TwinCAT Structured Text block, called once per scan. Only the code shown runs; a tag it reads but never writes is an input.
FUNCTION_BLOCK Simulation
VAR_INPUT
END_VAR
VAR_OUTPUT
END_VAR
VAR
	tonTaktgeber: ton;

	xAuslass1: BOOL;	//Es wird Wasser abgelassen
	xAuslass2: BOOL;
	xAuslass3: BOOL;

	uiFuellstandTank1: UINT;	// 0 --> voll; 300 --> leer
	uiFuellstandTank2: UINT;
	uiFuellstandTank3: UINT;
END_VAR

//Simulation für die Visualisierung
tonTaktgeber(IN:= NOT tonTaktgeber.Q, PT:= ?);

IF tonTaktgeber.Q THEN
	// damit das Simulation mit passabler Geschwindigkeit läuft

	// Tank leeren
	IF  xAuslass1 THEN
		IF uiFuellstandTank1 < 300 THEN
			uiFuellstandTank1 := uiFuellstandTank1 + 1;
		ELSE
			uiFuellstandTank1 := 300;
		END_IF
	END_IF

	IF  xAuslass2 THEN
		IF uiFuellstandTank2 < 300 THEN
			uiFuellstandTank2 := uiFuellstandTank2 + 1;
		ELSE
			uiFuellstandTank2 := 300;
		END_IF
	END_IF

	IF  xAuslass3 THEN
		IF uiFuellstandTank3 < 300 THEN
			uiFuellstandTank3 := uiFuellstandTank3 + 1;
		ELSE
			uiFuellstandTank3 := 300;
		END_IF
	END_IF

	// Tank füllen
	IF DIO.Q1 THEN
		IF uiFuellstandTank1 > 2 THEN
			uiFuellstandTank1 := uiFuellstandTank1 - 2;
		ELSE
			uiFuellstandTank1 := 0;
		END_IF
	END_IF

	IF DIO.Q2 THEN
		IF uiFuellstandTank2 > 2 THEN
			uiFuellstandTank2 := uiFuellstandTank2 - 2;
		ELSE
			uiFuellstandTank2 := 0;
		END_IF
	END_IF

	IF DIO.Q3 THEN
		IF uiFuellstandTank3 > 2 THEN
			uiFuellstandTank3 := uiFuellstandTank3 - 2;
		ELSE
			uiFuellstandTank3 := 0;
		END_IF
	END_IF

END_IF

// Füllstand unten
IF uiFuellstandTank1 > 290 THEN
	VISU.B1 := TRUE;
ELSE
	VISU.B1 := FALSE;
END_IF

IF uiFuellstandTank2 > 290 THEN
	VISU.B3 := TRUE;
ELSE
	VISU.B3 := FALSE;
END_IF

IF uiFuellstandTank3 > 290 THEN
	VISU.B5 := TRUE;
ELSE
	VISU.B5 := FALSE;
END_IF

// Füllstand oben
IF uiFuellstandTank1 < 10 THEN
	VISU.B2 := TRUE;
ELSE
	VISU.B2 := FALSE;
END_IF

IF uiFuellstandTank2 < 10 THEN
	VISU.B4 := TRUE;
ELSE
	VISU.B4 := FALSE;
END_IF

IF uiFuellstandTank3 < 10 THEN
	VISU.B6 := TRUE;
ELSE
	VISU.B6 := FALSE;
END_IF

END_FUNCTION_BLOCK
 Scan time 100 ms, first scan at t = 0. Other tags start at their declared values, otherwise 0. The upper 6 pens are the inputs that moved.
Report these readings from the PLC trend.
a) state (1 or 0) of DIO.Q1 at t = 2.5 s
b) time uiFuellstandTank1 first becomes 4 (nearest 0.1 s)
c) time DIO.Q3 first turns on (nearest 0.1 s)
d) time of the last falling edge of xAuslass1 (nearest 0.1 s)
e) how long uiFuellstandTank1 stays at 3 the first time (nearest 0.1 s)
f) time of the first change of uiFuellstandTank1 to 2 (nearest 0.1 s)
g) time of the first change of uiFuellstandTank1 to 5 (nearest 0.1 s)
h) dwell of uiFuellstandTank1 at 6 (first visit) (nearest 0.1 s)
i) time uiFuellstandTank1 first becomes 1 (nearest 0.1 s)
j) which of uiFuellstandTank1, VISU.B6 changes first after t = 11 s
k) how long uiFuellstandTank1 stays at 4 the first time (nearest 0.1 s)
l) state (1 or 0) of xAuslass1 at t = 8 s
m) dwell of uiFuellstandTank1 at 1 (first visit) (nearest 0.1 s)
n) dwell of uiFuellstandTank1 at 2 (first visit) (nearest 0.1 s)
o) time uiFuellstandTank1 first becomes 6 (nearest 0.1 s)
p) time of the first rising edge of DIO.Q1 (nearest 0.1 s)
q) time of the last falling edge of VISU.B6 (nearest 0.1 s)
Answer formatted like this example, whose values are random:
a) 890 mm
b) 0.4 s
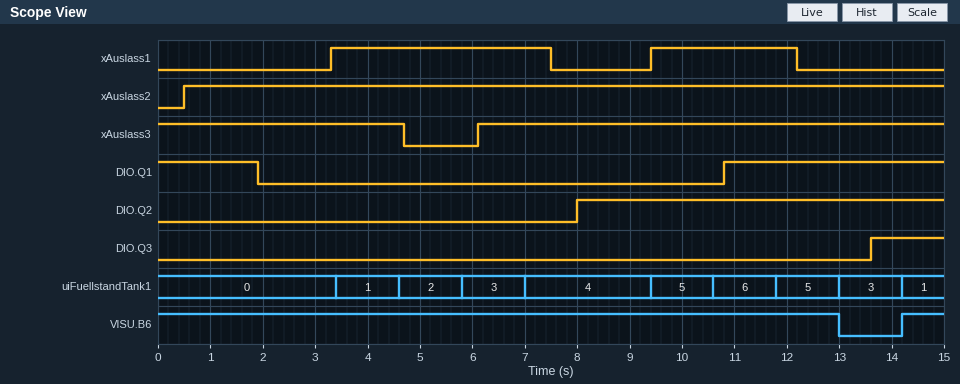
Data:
a) 0
b) 7.0 s
c) 13.6 s
d) 12.2 s
e) 1.2 s
f) 4.6 s
g) 9.4 s
h) 1.2 s
i) 3.4 s
j) uiFuellstandTank1
k) 2.4 s
l) 0
m) 1.2 s
n) 1.2 s
o) 10.6 s
p) 10.8 s
q) 13.0 s
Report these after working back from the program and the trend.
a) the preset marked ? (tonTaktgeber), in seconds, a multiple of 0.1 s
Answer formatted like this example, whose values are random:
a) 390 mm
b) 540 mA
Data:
a) 1.0 s
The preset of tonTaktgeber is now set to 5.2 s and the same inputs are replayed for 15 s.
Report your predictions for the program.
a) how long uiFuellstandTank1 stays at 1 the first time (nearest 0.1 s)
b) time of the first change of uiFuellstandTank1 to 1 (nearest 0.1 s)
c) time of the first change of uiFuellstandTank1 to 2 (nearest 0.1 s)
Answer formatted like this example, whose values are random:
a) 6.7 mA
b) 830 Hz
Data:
a) 5.4 s
b) 5.2 s
c) 10.6 s
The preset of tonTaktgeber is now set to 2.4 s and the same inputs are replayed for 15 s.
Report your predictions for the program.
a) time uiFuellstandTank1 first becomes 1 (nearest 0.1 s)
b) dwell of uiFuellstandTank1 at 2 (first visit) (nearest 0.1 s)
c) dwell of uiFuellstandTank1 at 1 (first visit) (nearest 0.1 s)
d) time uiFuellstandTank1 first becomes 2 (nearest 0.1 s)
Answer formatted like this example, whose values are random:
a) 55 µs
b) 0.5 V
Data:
a) 5.0 s
b) 2.6 s
c) 5.2 s
d) 10.2 s
